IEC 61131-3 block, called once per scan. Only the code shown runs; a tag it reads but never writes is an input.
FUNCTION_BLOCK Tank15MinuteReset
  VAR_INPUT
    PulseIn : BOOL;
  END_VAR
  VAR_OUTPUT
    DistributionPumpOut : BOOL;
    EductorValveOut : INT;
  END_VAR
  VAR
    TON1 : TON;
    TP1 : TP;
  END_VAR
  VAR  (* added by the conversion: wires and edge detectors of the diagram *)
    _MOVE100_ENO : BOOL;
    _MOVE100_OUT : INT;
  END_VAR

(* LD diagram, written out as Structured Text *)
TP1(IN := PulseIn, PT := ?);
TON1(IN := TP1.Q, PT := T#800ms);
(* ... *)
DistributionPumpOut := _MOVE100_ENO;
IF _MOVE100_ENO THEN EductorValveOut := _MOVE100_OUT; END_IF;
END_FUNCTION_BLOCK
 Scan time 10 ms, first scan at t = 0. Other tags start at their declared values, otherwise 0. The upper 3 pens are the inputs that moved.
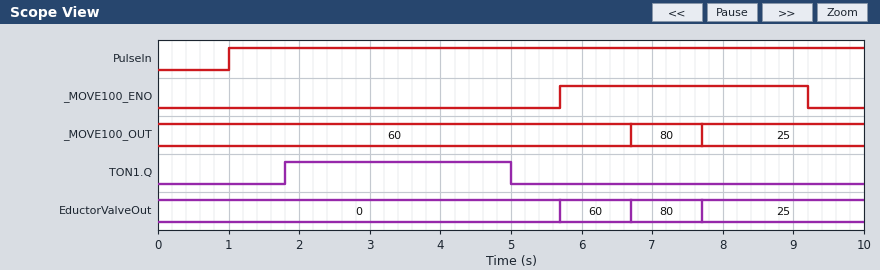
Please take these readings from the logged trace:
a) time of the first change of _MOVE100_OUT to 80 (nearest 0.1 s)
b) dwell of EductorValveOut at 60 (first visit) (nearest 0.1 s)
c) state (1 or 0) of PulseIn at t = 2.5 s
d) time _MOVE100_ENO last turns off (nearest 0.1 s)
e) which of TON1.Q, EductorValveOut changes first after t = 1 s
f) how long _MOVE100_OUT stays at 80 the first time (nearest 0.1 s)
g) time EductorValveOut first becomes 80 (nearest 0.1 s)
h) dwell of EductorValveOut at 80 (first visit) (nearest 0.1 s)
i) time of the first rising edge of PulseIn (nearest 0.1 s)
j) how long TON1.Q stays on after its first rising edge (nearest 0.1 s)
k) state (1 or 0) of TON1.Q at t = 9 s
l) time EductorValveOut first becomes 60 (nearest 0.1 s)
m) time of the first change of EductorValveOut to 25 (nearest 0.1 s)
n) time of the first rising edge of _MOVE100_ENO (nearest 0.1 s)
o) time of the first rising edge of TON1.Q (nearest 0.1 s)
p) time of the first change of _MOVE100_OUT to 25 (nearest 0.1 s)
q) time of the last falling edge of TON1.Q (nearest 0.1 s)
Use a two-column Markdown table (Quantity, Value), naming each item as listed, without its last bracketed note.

| Quantity | Value |
|---|---|
| time of the first change of _MOVE100_OUT to 80 | 6.7 s |
| dwell of EductorValveOut at 60 (first visit) | 1.0 s |
| state (1 or 0) of PulseIn at t = 2.5 s | 1 |
| time _MOVE100_ENO last turns off | 9.2 s |
| which of TON1.Q, EductorValveOut changes first after t = 1 s | TON1.Q |
| how long _MOVE100_OUT stays at 80 the first time | 1.0 s |
| time EductorValveOut first becomes 80 | 6.7 s |
| dwell of EductorValveOut at 80 (first visit) | 1.0 s |
| time of the first rising edge of PulseIn | 1.0 s |
| how long TON1.Q stays on after its first rising edge | 3.2 s |
| state (1 or 0) of TON1.Q at t = 9 s | 0 |
| time EductorValveOut first becomes 60 | 5.7 s |
| time of the first change of EductorValveOut to 25 | 7.7 s |
| time of the first rising edge of _MOVE100_ENO | 5.7 s |
| time of the first rising edge of TON1.Q | 1.8 s |
| time of the first change of _MOVE100_OUT to 25 | 7.7 s |
| time of the last falling edge of TON1.Q | 5.0 s |
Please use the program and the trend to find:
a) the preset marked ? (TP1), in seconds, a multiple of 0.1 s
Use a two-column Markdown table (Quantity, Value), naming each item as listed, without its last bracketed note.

| Quantity | Value |
|---|---|
| the preset marked ? (TP1), in seconds, a multiple of 0.1 s | 4.0 s |
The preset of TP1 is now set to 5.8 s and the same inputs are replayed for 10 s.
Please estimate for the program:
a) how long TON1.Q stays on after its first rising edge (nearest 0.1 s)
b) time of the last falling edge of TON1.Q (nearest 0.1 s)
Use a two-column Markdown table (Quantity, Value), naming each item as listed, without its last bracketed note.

| Quantity | Value |
|---|---|
| how long TON1.Q stays on after its first rising edge | 5.0 s |
| time of the last falling edge of TON1.Q | 6.8 s |
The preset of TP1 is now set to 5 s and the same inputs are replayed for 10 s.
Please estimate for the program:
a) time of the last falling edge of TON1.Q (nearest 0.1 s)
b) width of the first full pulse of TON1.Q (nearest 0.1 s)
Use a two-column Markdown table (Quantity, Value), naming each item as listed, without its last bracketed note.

| Quantity | Value |
|---|---|
| time of the last falling edge of TON1.Q | 6.0 s |
| width of the first full pulse of TON1.Q | 4.2 s |
